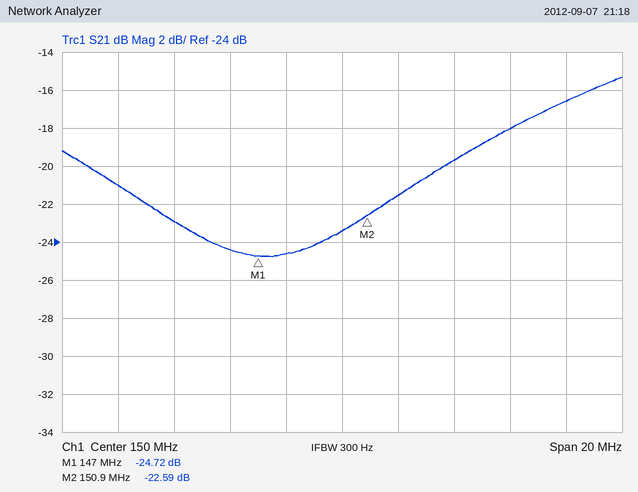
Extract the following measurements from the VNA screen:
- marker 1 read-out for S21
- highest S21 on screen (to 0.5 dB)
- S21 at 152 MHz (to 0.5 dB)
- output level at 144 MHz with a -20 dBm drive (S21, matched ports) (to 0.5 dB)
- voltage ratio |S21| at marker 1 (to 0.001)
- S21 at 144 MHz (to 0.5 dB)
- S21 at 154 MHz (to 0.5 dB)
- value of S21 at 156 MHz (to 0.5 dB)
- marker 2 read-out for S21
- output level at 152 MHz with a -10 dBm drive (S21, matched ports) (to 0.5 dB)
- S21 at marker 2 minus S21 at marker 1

-24.72 dB
-15.5 dB
-21.5 dB
-43.0 dBm
0.058
-23.0 dB
-19.5 dB
-18.0 dB
-22.59 dB
-31.5 dBm
2.13 dB
